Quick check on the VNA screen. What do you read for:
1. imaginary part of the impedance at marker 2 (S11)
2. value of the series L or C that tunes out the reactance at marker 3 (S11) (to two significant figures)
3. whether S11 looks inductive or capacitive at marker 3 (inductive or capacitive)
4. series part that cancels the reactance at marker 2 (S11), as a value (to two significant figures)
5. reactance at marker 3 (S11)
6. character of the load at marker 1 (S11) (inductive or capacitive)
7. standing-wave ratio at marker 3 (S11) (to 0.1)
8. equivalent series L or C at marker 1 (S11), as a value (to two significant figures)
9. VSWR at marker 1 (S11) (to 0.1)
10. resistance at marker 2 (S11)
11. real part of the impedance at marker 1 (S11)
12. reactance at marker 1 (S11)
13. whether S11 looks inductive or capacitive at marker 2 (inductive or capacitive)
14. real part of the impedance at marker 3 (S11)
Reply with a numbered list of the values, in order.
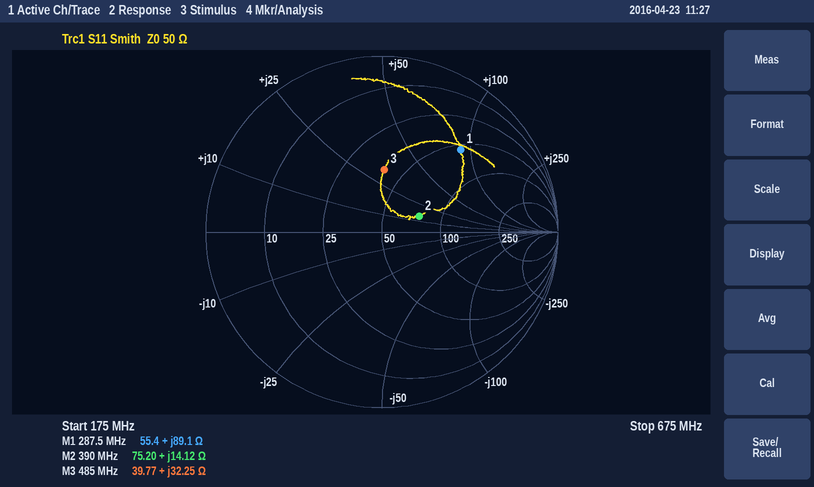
1. +14.12 Ω
2. 10 pF
3. inductive
4. 29 pF
5. +32.25 Ω
6. inductive
7. 2.1
8. 49 nH
9. 4.7
10. 75.20 Ω
11. 55.4 Ω
12. +89.1 Ω
13. inductive
14. 39.77 Ω
